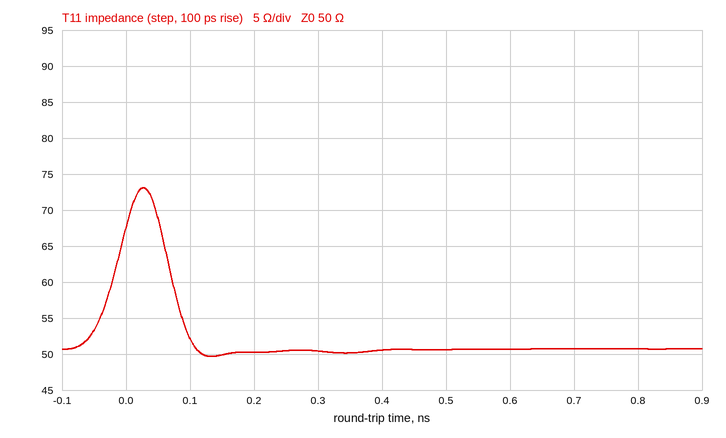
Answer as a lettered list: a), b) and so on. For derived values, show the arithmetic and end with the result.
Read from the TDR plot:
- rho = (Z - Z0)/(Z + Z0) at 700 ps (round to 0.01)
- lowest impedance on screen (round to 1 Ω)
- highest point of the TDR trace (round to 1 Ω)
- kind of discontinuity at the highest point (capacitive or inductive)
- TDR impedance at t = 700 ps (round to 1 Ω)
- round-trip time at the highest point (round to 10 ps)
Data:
a) (51 − 50)/(51 + 50) ≈ +0.01
b) 50 Ω
c) 73 Ω
d) inductive
e) 51 Ω
f) 30 ps
